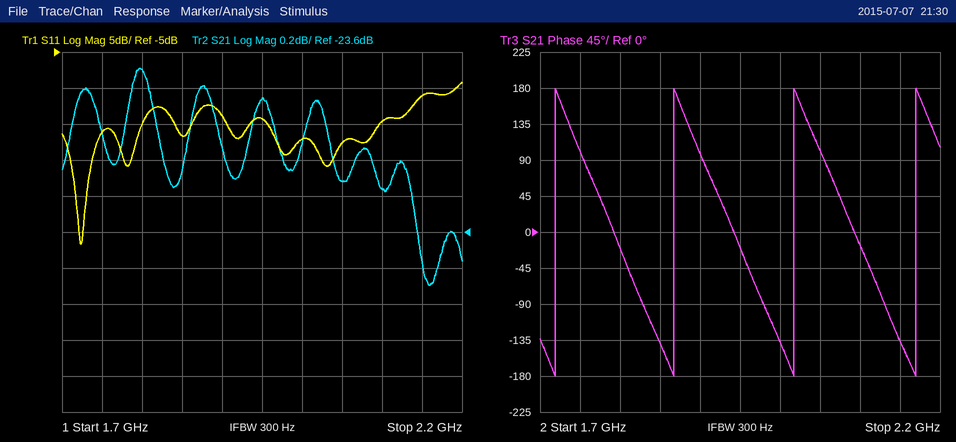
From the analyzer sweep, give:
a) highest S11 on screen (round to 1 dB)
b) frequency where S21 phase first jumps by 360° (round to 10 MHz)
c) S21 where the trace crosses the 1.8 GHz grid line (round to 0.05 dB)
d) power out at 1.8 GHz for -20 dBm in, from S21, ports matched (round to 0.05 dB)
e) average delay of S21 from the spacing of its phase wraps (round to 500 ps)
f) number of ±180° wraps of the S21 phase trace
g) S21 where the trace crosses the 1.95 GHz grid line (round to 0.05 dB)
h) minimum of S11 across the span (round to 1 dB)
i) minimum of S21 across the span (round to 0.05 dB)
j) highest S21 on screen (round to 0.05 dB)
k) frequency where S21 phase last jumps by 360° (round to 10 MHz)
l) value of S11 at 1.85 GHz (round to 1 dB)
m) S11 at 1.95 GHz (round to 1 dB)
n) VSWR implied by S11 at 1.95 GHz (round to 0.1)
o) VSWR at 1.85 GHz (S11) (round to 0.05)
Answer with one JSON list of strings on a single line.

["-9 dB", "1.72 GHz", "-22.70 dB", "-42.70 dBm", "6.5 ns", "4", "-22.85 dB", "-32 dB", "-23.90 dB", "-22.70 dB", "2.17 GHz", "-17 dB", "-14 dB", "1.5", "1.35"]
